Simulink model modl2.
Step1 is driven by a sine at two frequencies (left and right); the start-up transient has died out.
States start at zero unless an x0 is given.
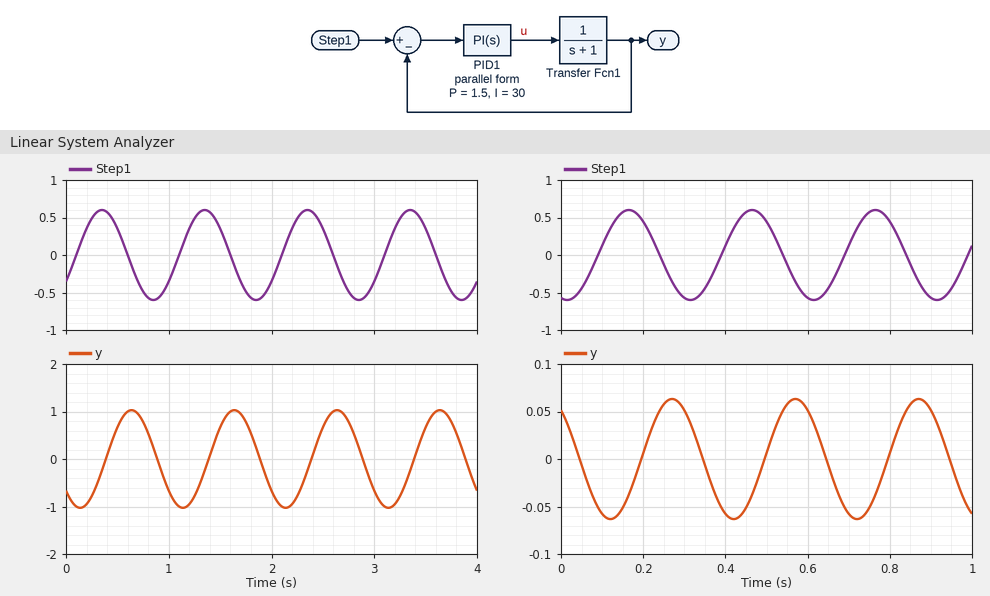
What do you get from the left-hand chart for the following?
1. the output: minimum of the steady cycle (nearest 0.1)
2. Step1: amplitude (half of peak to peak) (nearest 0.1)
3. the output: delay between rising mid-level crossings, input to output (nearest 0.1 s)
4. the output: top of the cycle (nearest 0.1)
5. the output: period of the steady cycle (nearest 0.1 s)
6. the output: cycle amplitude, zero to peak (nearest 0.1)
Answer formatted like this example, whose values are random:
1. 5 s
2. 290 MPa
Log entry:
1. -1.0
2. 0.6
3. 0.3 s
4. 1.0
5. 1.0 s
6. 1.0
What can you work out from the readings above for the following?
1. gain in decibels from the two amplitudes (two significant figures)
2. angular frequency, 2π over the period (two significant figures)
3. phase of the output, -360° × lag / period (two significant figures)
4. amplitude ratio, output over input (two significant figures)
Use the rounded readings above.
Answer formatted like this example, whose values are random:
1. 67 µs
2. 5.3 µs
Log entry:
1. 4.4 dB
2. 6.3 rad/s
3. -110°
4. 1.7
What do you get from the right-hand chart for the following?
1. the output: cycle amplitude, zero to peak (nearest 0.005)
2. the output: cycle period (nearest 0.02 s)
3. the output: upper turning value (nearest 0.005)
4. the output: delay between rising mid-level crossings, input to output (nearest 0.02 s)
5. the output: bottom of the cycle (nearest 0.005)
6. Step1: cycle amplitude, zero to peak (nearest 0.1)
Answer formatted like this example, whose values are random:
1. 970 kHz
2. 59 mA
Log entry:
1. 0.065
2. 0.30 s
3. 0.065
4. 0.10 s
5. -0.065
6. 0.6
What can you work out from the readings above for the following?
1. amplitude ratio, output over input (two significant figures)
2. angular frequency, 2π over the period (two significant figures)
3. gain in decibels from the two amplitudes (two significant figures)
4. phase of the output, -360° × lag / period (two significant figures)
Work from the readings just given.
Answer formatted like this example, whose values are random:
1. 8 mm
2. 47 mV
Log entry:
1. 0.11
2. 21 rad/s
3. -19 dB
4. -120°
